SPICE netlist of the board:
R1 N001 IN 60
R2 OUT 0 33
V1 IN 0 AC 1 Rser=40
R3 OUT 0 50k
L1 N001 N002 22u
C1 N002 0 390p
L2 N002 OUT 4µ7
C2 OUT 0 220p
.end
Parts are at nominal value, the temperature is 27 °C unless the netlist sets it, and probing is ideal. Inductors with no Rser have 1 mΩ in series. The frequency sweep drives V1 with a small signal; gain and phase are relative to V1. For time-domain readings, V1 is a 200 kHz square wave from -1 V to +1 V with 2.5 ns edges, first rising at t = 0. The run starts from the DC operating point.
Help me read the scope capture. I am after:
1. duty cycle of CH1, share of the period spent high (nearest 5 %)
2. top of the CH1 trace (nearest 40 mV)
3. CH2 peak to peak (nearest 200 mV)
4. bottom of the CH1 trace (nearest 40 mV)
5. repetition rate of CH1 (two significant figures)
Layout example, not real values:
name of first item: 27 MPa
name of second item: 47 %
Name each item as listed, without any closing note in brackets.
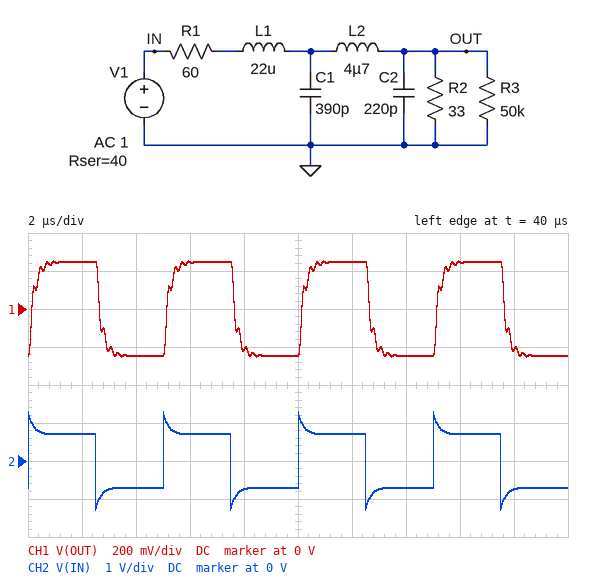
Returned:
duty cycle of CH1, share of the period spent high: 50 %
top of the CH1 trace: 240 mV
CH2 peak to peak: 2.6 V
bottom of the CH1 trace: -240 mV
repetition rate of CH1: 200 kHz
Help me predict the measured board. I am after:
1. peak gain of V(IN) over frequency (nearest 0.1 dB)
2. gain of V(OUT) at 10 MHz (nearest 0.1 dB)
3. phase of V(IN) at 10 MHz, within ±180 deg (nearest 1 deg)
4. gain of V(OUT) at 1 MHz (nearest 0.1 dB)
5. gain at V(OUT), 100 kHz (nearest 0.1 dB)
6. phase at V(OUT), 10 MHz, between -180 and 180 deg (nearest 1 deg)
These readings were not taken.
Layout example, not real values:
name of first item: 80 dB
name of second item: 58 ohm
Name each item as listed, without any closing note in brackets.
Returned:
peak gain of V(IN) over frequency: 0 dB
gain of V(OUT) at 10 MHz: -48.5 dB
phase of V(IN) at 10 MHz, within ±180 deg: 2 deg
gain of V(OUT) at 1 MHz: -15.7 dB
gain at V(OUT), 100 kHz: -12.2 dB
phase at V(OUT), 10 MHz, between -180 and 180 deg: 76 deg
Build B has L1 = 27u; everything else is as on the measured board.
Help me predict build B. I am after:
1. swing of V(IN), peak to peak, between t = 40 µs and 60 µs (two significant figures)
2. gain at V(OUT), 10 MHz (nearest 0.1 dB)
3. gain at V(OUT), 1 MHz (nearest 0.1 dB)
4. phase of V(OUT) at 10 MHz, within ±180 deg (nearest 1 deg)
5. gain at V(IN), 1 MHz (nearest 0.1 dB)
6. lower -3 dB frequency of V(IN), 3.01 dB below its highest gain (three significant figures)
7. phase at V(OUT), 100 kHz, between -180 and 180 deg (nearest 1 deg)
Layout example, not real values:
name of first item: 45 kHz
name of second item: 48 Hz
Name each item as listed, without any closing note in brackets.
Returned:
swing of V(IN), peak to peak, between t = 40 µs and 60 µs: 2.6 V
gain at V(OUT), 10 MHz: -50.3 dB
gain at V(OUT), 1 MHz: -16.7 dB
phase of V(OUT) at 10 MHz, within ±180 deg: 75 deg
gain at V(IN), 1 MHz: -0.8 dB
lower -3 dB frequency of V(IN), 3.01 dB below its highest gain: 101 kHz
phase at V(OUT), 100 kHz, between -180 and 180 deg: -9 deg
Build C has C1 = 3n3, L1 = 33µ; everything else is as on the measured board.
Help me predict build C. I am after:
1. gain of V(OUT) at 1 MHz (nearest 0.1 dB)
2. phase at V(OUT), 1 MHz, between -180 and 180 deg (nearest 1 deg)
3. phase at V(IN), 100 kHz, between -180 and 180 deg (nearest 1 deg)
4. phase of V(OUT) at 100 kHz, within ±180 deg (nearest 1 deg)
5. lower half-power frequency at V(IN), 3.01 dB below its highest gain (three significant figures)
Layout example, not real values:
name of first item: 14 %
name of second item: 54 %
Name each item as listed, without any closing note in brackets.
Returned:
gain of V(OUT) at 1 MHz: -15.4 dB
phase at V(OUT), 1 MHz, between -180 and 180 deg: -113 deg
phase at V(IN), 100 kHz, between -180 and 180 deg: 4 deg
phase of V(OUT) at 100 kHz, within ±180 deg: -13 deg
lower half-power frequency at V(IN), 3.01 dB below its highest gain: 90.8 kHz
